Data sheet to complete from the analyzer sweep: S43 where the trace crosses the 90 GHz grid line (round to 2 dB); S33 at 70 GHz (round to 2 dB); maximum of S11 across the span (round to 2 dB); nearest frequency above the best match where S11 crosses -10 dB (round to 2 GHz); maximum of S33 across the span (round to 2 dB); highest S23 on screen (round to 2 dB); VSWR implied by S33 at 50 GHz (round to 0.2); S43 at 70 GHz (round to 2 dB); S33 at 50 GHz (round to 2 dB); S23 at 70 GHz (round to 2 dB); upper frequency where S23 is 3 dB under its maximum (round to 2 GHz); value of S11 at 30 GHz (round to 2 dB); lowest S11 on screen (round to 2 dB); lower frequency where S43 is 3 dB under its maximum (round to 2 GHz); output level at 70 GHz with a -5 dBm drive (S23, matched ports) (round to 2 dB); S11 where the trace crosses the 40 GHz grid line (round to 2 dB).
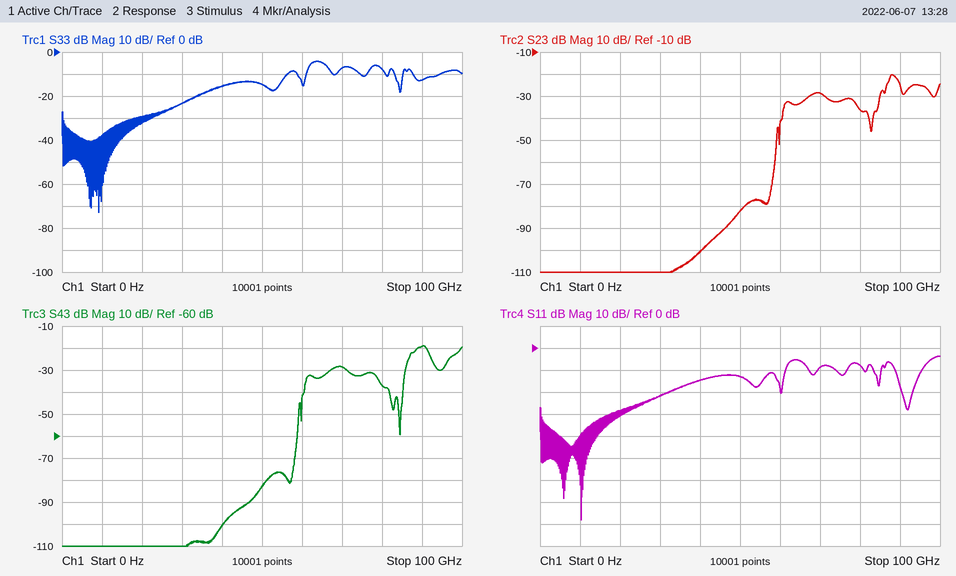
-20 dB
-8 dB
-4 dB
62 GHz
-4 dB
-20 dB
1.4
-28 dB
-14 dB
-28 dB
90 GHz
-22 dB
-78 dB
88 GHz
-34 dBm
-14 dB
